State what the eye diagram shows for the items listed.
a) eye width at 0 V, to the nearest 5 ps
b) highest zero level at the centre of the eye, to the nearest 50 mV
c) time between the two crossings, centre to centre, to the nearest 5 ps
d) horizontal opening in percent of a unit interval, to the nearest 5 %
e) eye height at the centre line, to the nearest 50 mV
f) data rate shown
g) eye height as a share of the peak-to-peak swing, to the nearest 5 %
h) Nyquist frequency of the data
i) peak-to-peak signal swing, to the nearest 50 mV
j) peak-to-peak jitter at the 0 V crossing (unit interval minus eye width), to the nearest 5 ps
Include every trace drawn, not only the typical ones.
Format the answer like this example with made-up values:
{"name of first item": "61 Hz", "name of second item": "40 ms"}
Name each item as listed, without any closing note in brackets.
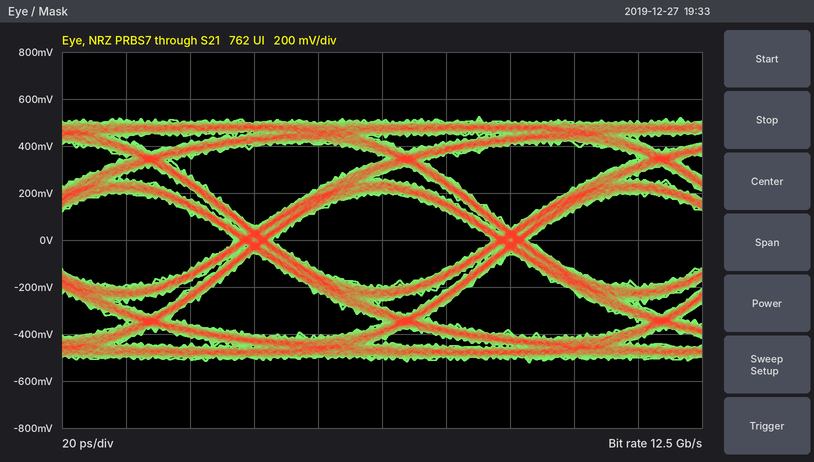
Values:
{"eye width at 0 V, to the nearest 5 ps": "70 ps", "highest zero level at the centre of the eye, to the nearest 50 mV": "-200 mV", "time between the two crossings, centre to centre, to the nearest 5 ps": "80 ps", "horizontal opening in percent of a unit interval, to the nearest 5 %": "85 %", "eye height at the centre line, to the nearest 50 mV": "400 mV", "data rate shown": "12.5 Gb/s", "eye height as a share of the peak-to-peak swing, to the nearest 5 %": "40 %", "Nyquist frequency of the data": "6.25 GHz", "peak-to-peak signal swing, to the nearest 50 mV": "1.05 V", "peak-to-peak jitter at the 0 V crossing (unit interval minus eye width), to the nearest 5 ps": "10 ps"}
